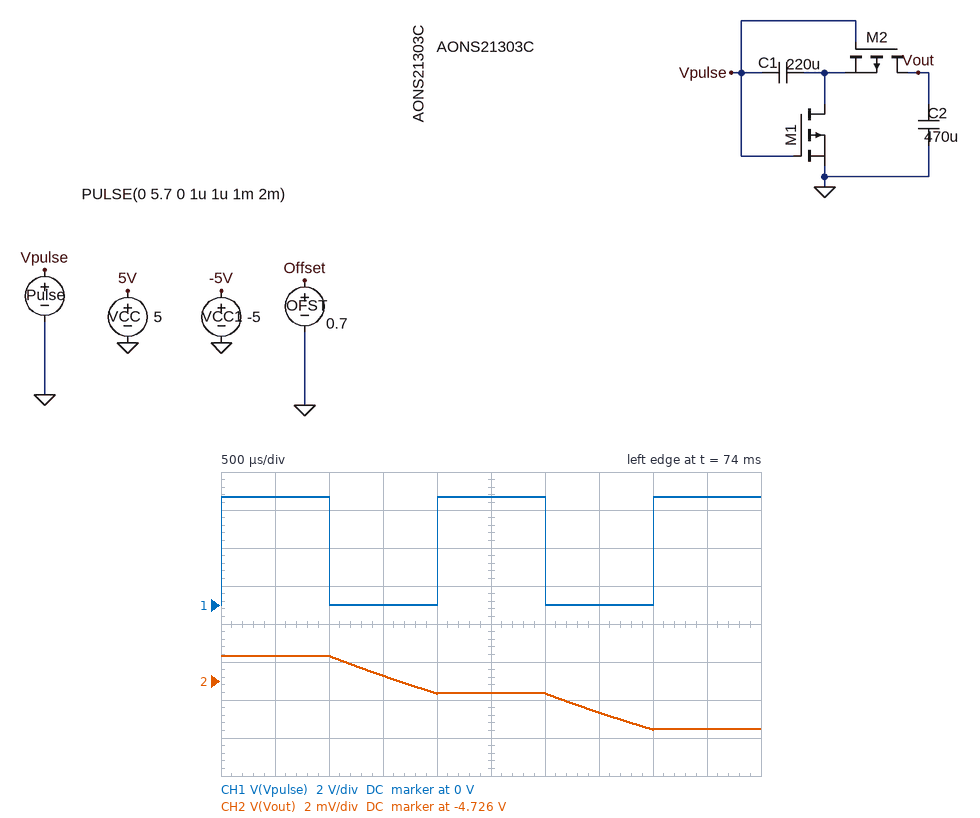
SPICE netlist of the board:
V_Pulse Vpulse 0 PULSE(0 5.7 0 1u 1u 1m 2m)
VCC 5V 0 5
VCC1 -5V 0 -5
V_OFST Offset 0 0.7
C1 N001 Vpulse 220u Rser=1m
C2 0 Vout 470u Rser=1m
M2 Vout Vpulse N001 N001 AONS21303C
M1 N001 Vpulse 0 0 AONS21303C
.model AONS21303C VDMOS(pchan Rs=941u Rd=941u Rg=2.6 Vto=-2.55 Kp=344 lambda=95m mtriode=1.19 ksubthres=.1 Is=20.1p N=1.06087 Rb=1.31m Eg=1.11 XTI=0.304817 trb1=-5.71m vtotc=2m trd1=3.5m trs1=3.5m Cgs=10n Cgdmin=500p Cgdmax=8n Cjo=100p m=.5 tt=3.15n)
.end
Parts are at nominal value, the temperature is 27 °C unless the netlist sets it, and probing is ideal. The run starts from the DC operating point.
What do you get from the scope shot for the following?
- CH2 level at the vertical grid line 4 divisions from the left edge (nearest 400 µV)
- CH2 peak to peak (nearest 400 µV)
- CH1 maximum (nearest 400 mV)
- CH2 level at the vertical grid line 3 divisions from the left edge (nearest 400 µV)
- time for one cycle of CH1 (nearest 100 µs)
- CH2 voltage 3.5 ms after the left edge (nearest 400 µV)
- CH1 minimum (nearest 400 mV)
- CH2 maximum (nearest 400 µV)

-4.7268 V
4.0 mV
5.6 V
-4.7256 V
2.0 ms
-4.7276 V
0 V
-4.7248 V
